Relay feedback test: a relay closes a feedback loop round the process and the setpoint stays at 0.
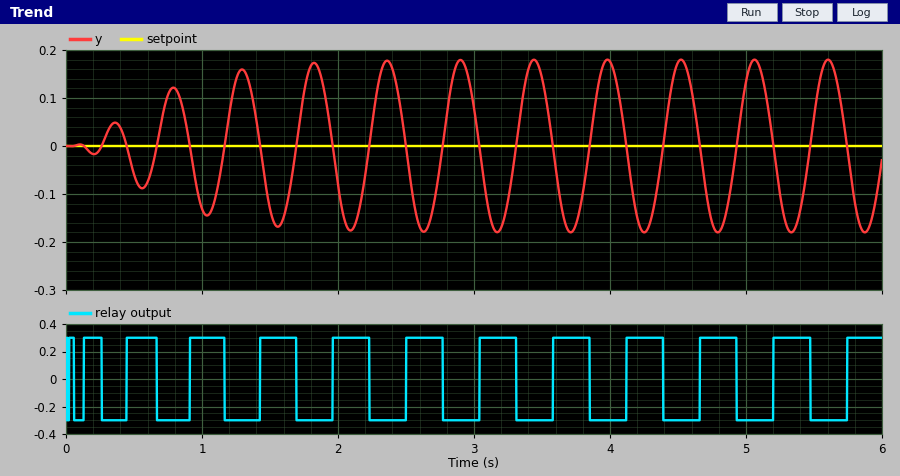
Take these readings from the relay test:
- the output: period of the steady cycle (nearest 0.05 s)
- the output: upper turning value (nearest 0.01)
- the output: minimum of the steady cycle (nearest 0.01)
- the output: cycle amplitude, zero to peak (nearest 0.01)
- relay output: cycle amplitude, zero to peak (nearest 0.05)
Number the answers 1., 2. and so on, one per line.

1. 0.55 s
2. 0.18
3. -0.18
4. 0.18
5. 0.30
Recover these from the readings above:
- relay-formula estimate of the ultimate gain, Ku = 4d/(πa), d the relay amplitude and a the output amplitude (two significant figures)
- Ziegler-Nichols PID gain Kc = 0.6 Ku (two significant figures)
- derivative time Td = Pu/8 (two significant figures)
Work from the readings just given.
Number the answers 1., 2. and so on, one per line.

1. 2.1
2. 1.3
3. 0.069 s
